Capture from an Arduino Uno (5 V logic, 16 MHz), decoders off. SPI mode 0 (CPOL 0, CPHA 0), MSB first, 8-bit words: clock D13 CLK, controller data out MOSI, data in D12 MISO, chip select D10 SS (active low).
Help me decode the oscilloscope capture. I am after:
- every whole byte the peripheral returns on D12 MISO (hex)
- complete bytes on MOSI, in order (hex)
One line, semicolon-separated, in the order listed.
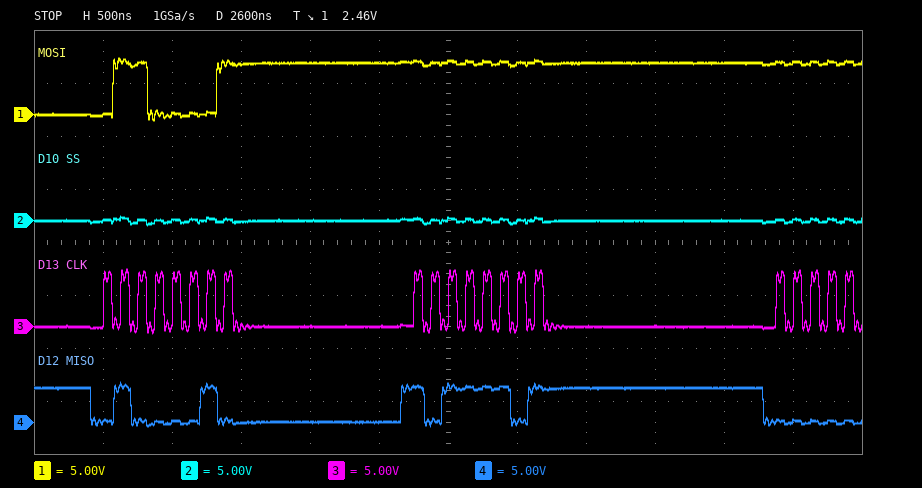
0x42 0xBD; 0x61 0xFF
